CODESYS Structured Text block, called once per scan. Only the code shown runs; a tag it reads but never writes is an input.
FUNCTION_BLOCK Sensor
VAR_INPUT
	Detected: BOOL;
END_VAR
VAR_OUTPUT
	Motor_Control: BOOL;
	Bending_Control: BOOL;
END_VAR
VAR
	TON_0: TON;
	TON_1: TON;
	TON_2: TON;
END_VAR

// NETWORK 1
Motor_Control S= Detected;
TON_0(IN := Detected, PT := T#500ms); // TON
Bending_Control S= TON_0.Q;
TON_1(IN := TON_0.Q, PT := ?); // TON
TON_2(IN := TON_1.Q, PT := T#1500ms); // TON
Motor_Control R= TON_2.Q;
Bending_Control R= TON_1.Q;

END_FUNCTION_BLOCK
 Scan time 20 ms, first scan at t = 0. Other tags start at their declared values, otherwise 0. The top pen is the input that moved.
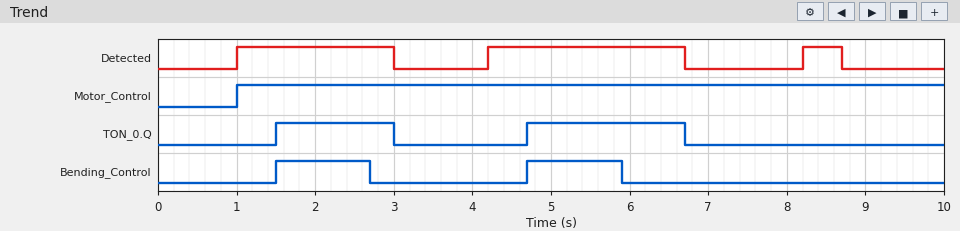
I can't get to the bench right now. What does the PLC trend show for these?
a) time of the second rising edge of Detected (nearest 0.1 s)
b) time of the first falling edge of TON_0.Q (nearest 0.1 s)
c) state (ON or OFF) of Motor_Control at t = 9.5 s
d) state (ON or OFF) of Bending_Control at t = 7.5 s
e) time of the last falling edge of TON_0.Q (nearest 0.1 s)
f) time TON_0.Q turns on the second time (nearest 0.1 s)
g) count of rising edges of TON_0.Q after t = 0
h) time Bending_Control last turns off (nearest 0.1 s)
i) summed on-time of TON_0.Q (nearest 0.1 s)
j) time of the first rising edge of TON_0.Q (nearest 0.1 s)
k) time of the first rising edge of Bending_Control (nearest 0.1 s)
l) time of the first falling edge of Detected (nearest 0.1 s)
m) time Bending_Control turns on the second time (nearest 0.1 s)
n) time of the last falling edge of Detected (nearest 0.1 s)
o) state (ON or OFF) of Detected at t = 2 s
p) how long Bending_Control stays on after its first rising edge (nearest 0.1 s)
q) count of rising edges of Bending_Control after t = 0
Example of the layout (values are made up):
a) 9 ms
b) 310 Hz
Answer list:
a) 4.2 s
b) 3.0 s
c) ON
d) OFF
e) 6.7 s
f) 4.7 s
g) 2
h) 5.9 s
i) 3.5 s
j) 1.5 s
k) 1.5 s
l) 3.0 s
m) 4.7 s
n) 8.7 s
o) ON
p) 1.2 s
q) 2
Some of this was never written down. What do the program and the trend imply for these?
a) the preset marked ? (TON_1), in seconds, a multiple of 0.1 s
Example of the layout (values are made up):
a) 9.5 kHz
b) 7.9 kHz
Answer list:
a) 1.2 s
